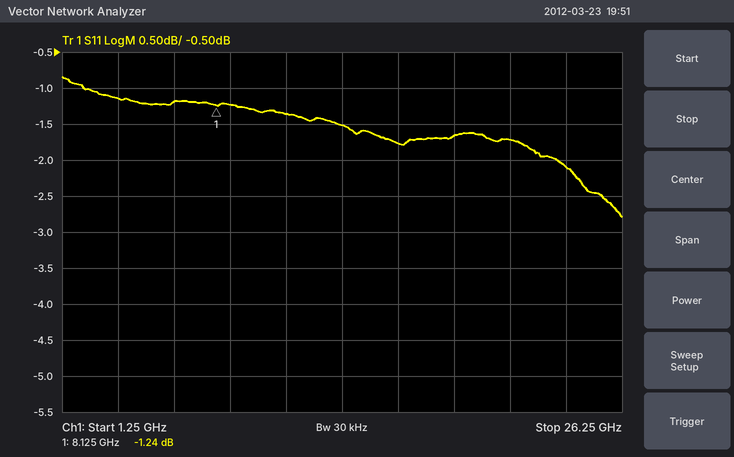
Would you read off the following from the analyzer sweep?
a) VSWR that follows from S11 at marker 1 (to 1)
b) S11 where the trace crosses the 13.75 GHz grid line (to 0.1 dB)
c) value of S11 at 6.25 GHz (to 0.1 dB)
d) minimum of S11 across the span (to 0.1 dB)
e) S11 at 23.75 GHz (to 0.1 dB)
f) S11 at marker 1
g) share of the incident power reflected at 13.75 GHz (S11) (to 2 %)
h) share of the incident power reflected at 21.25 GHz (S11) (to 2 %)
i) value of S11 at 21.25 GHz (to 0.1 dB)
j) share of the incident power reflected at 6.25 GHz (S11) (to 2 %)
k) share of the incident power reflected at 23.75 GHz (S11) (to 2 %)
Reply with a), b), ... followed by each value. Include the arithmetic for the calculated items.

a) (1 + 0.8670)/(1 − 0.8670) ≈ 14
b) -1.5 dB
c) -1.2 dB
d) -2.8 dB
e) -2.1 dB
f) -1.24 dB
g) 10^(-1.5/10) ≈ 70.8 %, so 70 % to the nearest 2 %
h) 10^(-1.7/10) ≈ 68 %
i) -1.7 dB
j) 10^(-1.2/10) ≈ 76 %
k) 10^(-2.1/10) ≈ 62 %
